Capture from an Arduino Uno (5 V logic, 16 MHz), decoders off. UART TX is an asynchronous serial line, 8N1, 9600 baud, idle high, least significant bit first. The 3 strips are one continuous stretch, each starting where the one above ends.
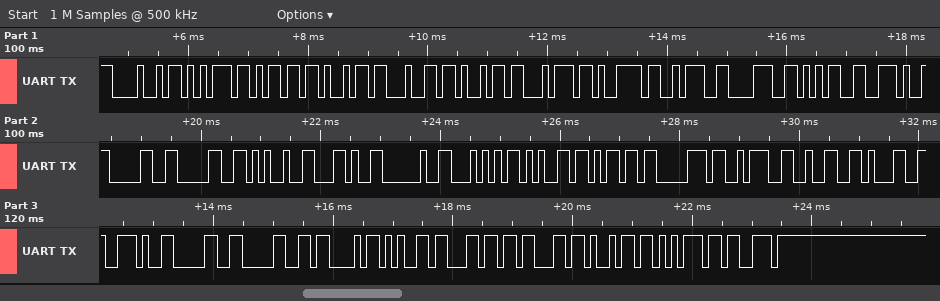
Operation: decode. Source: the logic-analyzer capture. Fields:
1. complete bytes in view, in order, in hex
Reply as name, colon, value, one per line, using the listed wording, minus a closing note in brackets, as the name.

complete bytes in view, in order, in hex: 48 75 6D 69 64 69 74 79 3A 38 35 2E 30 30 25 2C 20 54 65 6D 70 3A 32 31 2E 30 30 43 65 6C 63 69 75 73
